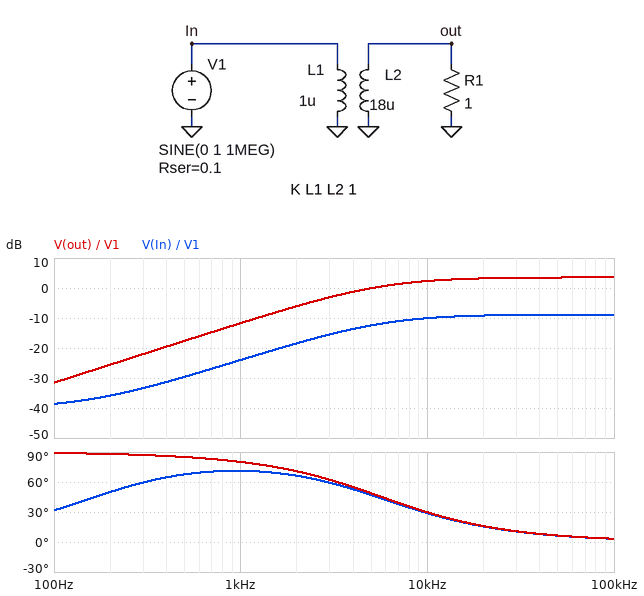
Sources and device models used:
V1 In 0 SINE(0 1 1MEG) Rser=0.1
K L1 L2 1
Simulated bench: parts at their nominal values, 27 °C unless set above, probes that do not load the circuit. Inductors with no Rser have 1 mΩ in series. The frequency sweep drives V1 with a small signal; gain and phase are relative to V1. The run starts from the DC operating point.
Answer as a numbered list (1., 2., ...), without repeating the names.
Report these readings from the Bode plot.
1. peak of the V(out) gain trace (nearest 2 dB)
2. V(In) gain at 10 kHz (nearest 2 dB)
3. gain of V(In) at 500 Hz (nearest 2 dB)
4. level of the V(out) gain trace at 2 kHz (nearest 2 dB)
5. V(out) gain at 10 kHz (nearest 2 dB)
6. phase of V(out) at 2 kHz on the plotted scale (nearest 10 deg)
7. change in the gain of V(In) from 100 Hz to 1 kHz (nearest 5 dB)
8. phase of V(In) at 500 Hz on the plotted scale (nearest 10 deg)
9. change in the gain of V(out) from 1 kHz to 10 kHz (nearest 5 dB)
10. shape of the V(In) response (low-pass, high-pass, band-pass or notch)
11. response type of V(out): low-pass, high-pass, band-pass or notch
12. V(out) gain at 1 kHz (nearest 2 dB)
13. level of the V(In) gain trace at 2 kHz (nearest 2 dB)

1. 4 dB
2. -10 dB
3. -30 dB
4. -6 dB
5. 2 dB
6. 70 deg
7. 15 dB
8. 70 deg
9. 15 dB
10. high-pass
11. high-pass
12. -12 dB
13. -18 dB
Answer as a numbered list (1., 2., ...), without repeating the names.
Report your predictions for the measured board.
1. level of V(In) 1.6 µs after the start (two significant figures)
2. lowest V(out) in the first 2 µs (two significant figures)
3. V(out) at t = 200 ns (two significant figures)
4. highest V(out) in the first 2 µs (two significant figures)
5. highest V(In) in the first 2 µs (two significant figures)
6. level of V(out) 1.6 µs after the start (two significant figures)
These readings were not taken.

1. -220 mV
2. -1.5 V
3. 1.4 V
4. 1.5 V
5. 360 mV
6. -900 mV
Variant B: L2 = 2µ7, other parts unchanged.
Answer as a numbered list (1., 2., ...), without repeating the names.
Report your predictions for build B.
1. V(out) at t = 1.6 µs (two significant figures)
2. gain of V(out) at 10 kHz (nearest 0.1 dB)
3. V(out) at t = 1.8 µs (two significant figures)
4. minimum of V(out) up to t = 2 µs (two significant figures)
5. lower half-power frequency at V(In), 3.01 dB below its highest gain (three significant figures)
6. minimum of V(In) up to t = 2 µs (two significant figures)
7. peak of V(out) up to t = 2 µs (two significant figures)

1. -790 mV
2. -1.9 dB
3. -1.2 V
4. -1.3 V
5. 12.6 kHz
6. -800 mV
7. 1.3 V
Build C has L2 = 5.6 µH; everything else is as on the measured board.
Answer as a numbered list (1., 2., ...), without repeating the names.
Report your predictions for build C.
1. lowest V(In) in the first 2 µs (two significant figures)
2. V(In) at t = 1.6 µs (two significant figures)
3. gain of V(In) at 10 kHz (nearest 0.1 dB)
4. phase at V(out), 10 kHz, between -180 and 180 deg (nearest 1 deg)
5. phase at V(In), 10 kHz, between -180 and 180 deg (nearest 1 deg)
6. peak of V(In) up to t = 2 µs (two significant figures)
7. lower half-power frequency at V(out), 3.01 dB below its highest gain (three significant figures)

1. -650 mV
2. -390 mV
3. -7.0 dB
4. 46 deg
5. 45 deg
6. 640 mV
7. 10.3 kHz
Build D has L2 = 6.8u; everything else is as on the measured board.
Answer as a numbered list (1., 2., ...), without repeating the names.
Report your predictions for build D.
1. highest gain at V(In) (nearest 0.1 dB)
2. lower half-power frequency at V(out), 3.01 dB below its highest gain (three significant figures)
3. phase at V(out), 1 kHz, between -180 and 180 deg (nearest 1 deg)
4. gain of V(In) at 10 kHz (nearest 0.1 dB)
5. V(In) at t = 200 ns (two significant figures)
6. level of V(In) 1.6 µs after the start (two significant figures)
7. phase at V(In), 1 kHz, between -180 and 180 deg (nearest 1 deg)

1. -4.5 dB
2. 9.53 kHz
3. 84 deg
4. -7.3 dB
5. 560 mV
6. -360 mV
7. 75 deg
